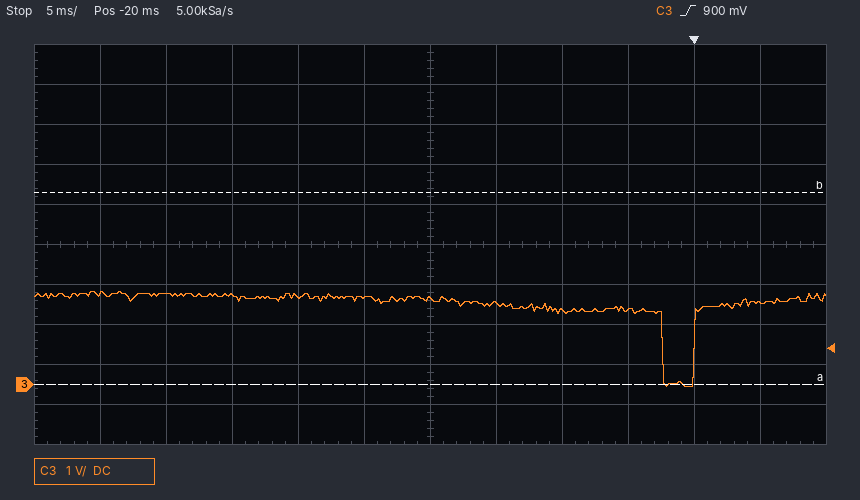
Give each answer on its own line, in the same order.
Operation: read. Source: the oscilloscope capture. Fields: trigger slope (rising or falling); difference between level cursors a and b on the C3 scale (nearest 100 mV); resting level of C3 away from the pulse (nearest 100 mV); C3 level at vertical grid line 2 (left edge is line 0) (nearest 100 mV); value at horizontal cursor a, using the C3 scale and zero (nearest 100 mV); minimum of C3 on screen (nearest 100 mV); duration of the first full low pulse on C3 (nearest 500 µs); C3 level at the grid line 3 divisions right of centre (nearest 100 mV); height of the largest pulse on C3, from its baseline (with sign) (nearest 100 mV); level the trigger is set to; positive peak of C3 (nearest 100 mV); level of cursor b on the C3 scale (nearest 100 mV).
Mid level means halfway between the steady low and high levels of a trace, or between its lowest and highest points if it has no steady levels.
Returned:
rising
4.8 V
2.2 V
2.3 V
0.0 V
0.0 V
2.5 ms
1.9 V
-2.2 V
900 mV
2.3 V
4.8 V
